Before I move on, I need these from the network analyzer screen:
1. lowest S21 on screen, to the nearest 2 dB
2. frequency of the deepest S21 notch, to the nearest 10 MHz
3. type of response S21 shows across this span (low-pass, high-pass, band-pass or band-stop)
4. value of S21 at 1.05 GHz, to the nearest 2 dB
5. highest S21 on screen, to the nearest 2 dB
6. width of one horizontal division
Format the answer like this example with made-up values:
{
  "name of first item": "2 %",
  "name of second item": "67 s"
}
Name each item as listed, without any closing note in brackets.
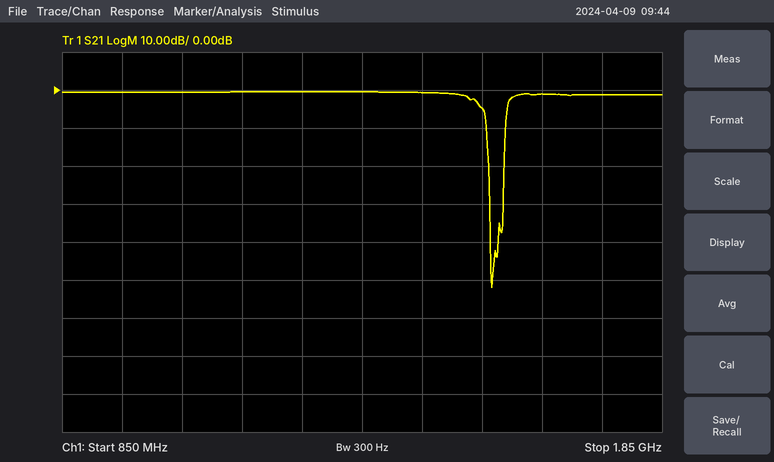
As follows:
{
  "lowest S21 on screen, to the nearest 2 dB": "-52 dB",
  "frequency of the deepest S21 notch, to the nearest 10 MHz": "1.57 GHz",
  "type of response S21 shows across this span": "band-stop",
  "value of S21 at 1.05 GHz, to the nearest 2 dB": "0 dB",
  "highest S21 on screen, to the nearest 2 dB": "0 dB",
  "width of one horizontal division": "100 MHz"
}
